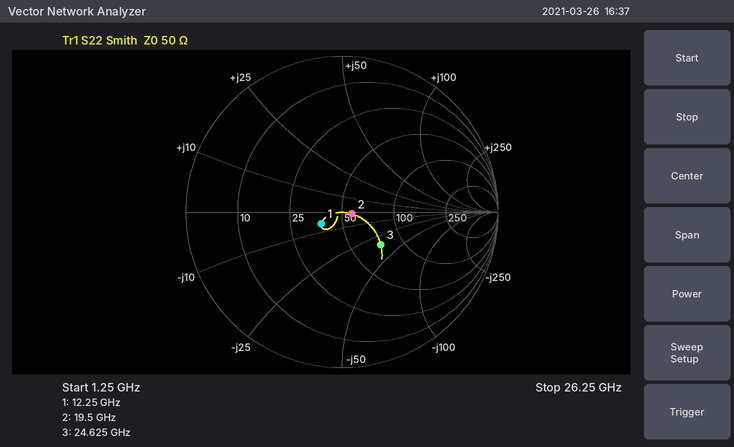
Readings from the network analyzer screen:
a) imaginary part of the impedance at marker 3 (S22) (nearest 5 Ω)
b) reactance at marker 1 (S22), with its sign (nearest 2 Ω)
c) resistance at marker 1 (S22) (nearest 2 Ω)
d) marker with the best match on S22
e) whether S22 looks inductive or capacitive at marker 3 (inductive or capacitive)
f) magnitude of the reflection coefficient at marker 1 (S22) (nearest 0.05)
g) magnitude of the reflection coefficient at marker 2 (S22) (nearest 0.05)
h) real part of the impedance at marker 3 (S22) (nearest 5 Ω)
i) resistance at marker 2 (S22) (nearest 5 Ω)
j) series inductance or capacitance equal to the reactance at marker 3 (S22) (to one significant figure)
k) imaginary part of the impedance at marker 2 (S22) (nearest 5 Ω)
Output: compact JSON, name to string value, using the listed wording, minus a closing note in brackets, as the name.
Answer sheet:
{"imaginary part of the impedance at marker 3 (S22)": "-35 Ω", "reactance at marker 1 (S22), with its sign": "-6 Ω", "resistance at marker 1 (S22)": "38 Ω", "marker with the best match on S22": "marker 2", "whether S22 looks inductive or capacitive at marker 3": "capacitive", "magnitude of the reflection coefficient at marker 1 (S22)": "0.15", "magnitude of the reflection coefficient at marker 2 (S22)": "0.05", "real part of the impedance at marker 3 (S22)": "75 Ω", "resistance at marker 2 (S22)": "55 Ω", "series inductance or capacitance equal to the reactance at marker 3 (S22)": "200 fF", "imaginary part of the impedance at marker 2 (S22)": "0 Ω"}
